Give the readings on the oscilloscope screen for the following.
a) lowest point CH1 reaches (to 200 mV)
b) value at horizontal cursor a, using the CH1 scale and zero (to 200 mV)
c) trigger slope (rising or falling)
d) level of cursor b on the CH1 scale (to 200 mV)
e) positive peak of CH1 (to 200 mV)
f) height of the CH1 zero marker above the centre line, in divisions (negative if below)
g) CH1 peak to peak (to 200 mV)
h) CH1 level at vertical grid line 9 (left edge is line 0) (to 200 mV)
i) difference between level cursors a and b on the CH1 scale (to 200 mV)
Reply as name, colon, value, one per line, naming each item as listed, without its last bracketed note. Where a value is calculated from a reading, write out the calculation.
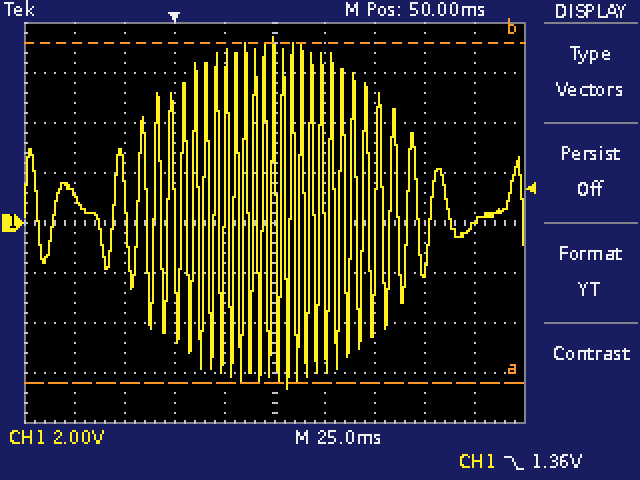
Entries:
lowest point CH1 reaches: -6.6 V
value at horizontal cursor a, using the CH1 scale and zero: -6.4 V
trigger slope: falling
level of cursor b on the CH1 scale: 7.2 V
positive peak of CH1: 7.4 V
height of the CH1 zero marker above the centre line, in divisions: 0.0 div
CH1 peak to peak: 7.4 V − (-6.6 V) = 14.0 V
CH1 level at vertical grid line 9 (left edge is line 0): 0.0 V
difference between level cursors a and b on the CH1 scale: 13.6 V
